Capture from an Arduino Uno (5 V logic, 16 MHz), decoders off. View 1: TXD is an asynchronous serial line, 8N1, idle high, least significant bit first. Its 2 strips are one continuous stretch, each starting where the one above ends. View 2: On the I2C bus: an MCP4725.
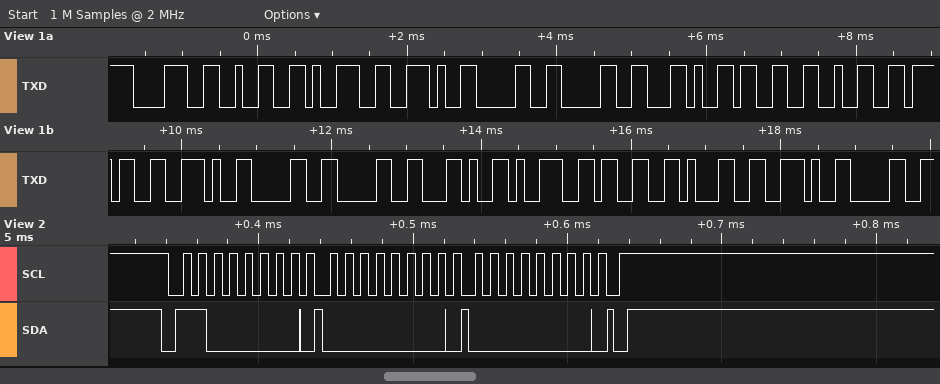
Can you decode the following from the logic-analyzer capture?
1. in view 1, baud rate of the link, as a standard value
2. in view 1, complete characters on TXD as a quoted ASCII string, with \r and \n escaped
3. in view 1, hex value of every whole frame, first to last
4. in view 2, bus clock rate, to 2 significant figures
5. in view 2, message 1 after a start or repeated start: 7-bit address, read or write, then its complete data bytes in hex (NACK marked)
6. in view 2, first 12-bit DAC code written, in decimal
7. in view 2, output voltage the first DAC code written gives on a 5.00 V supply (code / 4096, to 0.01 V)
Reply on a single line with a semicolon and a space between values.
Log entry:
9600 baud; "829.00,327.00,931.0"; 38 32 39 2E 30 30 2C 33 32 37 2E 30 30 2C 39 33 31 2E 30; 100 kHz; 0x60 write: 00 00; 0; 0.00 V
